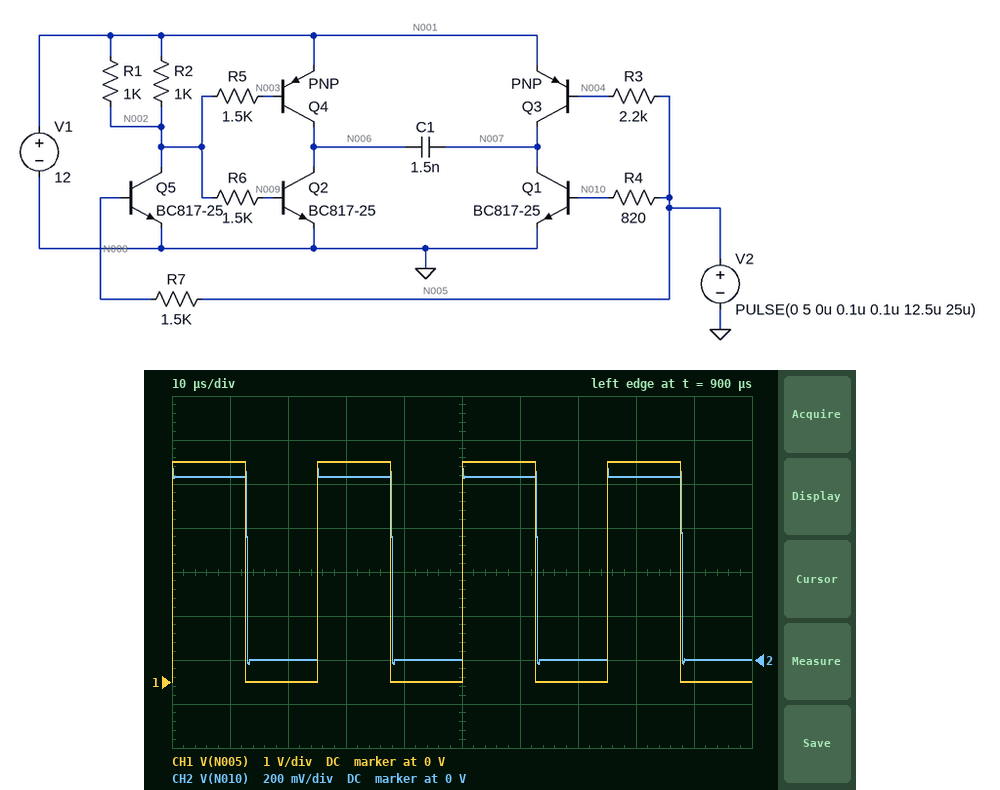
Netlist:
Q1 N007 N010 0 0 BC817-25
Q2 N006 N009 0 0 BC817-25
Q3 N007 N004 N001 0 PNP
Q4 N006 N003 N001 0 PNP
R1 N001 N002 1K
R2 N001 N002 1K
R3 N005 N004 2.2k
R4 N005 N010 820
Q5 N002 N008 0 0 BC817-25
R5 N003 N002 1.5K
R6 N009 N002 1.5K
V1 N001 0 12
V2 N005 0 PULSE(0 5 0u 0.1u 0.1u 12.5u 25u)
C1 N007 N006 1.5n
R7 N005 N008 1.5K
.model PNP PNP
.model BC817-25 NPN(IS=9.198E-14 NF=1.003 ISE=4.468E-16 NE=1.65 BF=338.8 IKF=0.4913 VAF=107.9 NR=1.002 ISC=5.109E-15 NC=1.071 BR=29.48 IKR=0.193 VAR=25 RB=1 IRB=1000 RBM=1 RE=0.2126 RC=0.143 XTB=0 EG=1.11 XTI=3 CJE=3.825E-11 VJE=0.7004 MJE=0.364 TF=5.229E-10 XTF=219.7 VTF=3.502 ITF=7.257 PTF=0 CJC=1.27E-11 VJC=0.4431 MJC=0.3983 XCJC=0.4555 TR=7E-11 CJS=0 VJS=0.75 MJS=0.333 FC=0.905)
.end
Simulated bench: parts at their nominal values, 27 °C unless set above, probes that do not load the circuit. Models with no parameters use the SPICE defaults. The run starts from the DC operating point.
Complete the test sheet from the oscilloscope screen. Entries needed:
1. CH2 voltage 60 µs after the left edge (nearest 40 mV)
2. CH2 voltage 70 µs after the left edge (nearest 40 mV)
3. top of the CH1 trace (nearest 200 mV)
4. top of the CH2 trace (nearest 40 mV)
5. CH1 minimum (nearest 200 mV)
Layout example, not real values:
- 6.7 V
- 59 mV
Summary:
- 840 mV
- 0 V
- 5.0 V
- 880 mV
- 0 V
